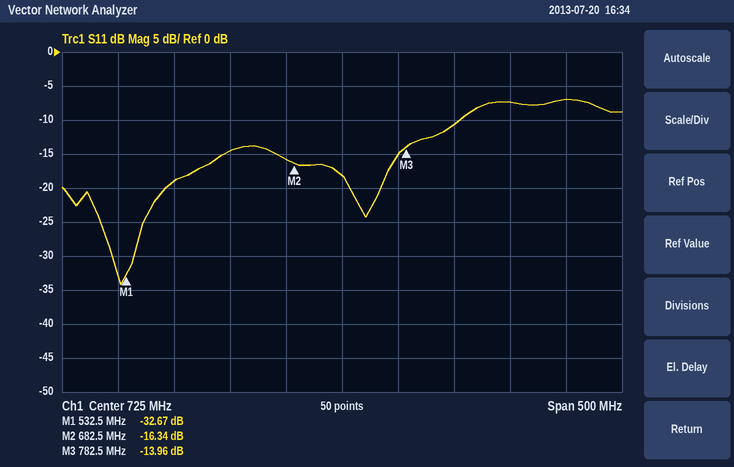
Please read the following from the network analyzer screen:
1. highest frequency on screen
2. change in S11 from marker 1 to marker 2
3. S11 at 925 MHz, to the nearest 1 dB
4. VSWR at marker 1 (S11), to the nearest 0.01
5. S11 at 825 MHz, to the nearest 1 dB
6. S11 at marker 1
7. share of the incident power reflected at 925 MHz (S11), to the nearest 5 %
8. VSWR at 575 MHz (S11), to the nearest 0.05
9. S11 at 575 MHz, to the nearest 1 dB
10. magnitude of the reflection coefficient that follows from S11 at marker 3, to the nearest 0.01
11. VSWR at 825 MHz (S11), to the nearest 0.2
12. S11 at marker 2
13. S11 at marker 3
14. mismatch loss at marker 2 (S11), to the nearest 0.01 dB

975 MHz
16.33 dB
-7 dB
1.05
-11 dB
-32.67 dB
20 %
1.25
-19 dB
0.20
1.8
-16.34 dB
-13.96 dB
0.10 dB
